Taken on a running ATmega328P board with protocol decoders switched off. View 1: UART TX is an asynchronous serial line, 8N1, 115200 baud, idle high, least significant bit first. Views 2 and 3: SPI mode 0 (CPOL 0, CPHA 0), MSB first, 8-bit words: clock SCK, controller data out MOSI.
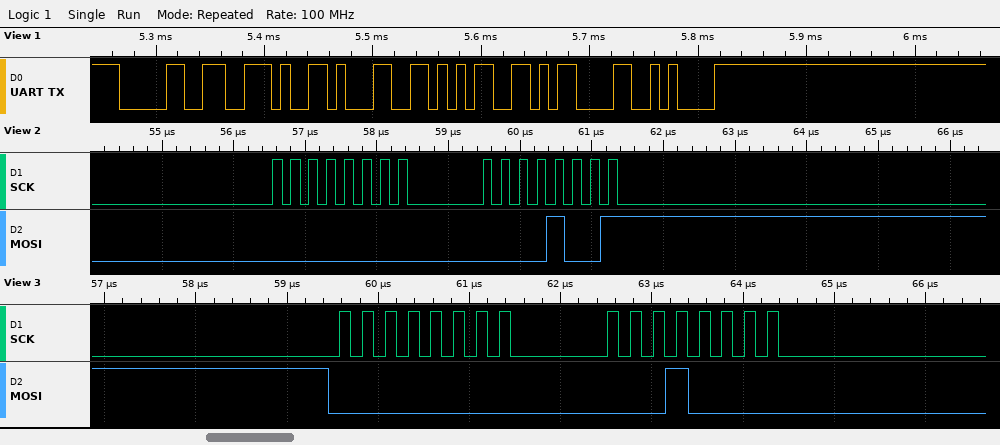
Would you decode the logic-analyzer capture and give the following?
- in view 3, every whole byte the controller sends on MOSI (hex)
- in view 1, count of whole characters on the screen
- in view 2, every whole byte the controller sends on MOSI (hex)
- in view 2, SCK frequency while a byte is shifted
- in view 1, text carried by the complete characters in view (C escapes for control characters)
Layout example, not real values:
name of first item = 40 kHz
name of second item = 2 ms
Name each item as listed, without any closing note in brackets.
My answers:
in view 3, every whole byte the controller sends on MOSI = 00 10
in view 1, count of whole characters on the screen = 6
in view 2, every whole byte the controller sends on MOSI = 0x00 0x09
in view 2, SCK frequency while a byte is shifted = 4 MHz
in view 1, text carried by the complete characters in view = "0.15\r\n"
